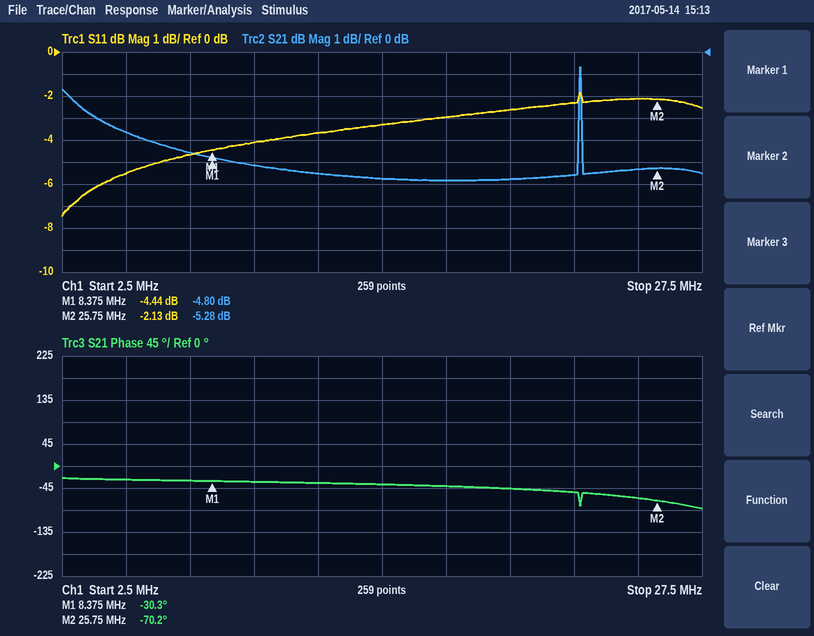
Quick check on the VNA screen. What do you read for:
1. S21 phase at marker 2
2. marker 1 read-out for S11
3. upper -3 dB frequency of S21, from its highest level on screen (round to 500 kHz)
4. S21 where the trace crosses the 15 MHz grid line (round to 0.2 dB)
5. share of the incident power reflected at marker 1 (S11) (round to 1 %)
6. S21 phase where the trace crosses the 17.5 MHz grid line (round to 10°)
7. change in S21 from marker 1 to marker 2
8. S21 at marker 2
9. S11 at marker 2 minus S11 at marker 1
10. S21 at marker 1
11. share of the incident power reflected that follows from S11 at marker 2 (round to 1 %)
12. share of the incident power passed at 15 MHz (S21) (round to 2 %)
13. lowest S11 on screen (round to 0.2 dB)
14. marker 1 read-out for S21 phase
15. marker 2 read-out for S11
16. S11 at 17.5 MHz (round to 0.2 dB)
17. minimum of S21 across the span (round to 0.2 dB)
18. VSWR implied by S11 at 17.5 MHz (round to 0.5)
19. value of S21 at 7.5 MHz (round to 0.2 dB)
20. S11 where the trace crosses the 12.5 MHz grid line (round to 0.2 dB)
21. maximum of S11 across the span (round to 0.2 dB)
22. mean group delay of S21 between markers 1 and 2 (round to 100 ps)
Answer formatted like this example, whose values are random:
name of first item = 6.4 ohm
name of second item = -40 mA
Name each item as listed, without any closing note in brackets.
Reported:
S21 phase at marker 2 = -70.2°
marker 1 read-out for S11 = -4.44 dB
upper -3 dB frequency of S21, from its highest level on screen = 23.0 MHz
S21 where the trace crosses the 15 MHz grid line = -5.8 dB
share of the incident power reflected at marker 1 (S11) = 36 %
S21 phase where the trace crosses the 17.5 MHz grid line = -40°
change in S21 from marker 1 to marker 2 = -0.48 dB
S21 at marker 2 = -5.28 dB
S11 at marker 2 minus S11 at marker 1 = 2.31 dB
S21 at marker 1 = -4.80 dB
share of the incident power reflected that follows from S11 at marker 2 = 61 %
share of the incident power passed at 15 MHz (S21) = 26 %
lowest S11 on screen = -7.4 dB
marker 1 read-out for S21 phase = -30.3°
marker 2 read-out for S11 = -2.13 dB
S11 at 17.5 MHz = -3.0 dB
minimum of S21 across the span = -5.8 dB
VSWR implied by S11 at 17.5 MHz = 6.0
value of S21 at 7.5 MHz = -4.6 dB
S11 where the trace crosses the 12.5 MHz grid line = -3.6 dB
maximum of S11 across the span = -1.8 dB
mean group delay of S21 between markers 1 and 2 = 6.4 ns
